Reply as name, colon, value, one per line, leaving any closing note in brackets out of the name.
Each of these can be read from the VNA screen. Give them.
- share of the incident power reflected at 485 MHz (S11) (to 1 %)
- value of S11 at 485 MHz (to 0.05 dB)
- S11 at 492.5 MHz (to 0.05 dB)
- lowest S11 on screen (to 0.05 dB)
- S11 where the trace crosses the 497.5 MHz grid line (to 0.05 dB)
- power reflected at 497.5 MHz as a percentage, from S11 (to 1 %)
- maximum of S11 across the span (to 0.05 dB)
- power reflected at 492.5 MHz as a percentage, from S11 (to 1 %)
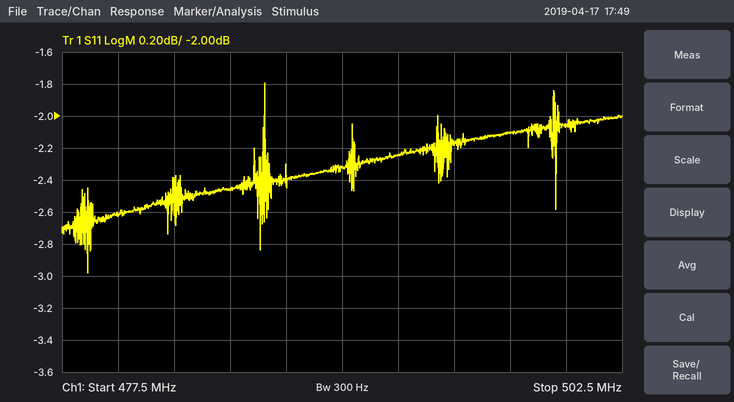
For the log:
share of the incident power reflected at 485 MHz (S11): 57 %
value of S11 at 485 MHz: -2.45 dB
S11 at 492.5 MHz: -2.25 dB
lowest S11 on screen: -3.00 dB
S11 where the trace crosses the 497.5 MHz grid line: -2.10 dB
power reflected at 497.5 MHz as a percentage, from S11: 62 %
maximum of S11 across the span: -1.80 dB
power reflected at 492.5 MHz as a percentage, from S11: 60 %
